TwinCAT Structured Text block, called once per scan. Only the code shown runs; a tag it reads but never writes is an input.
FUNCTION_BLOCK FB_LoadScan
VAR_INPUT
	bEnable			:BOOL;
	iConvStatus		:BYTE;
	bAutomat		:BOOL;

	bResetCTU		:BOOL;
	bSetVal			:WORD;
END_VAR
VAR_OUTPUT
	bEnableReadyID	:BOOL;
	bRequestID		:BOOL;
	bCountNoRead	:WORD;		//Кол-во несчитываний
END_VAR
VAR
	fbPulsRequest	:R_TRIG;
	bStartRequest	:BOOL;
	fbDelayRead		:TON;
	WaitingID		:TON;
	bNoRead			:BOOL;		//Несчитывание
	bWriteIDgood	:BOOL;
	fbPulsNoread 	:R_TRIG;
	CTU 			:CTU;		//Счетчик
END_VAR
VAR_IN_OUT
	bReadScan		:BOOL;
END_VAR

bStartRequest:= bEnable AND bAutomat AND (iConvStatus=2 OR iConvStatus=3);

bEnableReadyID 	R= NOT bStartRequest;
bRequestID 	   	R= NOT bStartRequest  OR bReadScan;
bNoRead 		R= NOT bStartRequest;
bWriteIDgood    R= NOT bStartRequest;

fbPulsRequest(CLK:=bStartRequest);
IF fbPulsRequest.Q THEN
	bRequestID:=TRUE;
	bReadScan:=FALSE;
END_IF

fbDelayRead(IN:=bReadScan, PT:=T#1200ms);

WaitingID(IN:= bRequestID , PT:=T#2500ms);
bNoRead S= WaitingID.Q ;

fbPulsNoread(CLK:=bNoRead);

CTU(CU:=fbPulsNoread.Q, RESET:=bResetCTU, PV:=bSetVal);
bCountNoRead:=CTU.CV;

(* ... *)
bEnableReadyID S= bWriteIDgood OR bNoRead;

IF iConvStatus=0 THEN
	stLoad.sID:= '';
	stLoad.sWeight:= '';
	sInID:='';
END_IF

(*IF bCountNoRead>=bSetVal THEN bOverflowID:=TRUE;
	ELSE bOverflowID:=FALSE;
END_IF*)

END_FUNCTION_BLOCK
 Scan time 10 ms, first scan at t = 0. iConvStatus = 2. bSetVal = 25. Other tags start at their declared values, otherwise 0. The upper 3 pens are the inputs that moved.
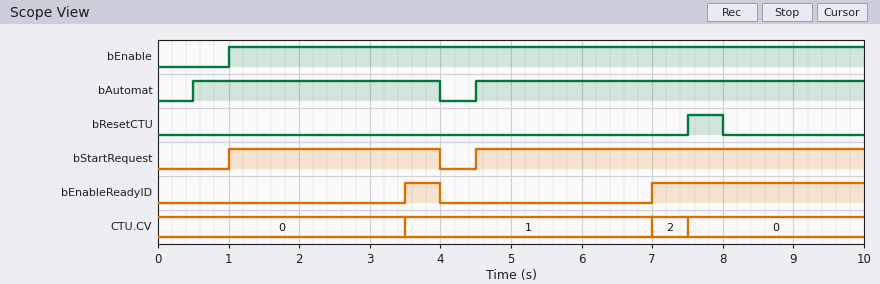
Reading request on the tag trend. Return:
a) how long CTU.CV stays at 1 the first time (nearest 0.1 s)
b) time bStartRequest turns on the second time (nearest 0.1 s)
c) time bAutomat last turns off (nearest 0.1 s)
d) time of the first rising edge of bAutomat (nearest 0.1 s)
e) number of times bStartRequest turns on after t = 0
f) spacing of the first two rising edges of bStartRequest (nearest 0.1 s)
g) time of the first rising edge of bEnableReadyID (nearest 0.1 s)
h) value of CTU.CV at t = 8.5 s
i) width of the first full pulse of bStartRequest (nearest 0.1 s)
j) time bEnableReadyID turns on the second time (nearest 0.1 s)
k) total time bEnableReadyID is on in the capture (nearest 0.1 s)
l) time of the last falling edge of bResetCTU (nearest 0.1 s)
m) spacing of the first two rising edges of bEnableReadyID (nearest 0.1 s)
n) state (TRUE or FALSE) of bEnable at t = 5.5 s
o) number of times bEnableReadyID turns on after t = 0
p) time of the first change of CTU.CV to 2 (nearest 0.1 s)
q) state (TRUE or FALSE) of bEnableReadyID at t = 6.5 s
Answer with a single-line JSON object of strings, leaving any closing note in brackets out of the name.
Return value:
{"how long CTU.CV stays at 1 the first time": "3.5 s", "time bStartRequest turns on the second time": "4.5 s", "time bAutomat last turns off": "4.0 s", "time of the first rising edge of bAutomat": "0.5 s", "number of times bStartRequest turns on after t = 0": "2", "spacing of the first two rising edges of bStartRequest": "3.5 s", "time of the first rising edge of bEnableReadyID": "3.5 s", "value of CTU.CV at t = 8.5 s": "0", "width of the first full pulse of bStartRequest": "3.0 s", "time bEnableReadyID turns on the second time": "7.0 s", "total time bEnableReadyID is on in the capture": "3.5 s", "time of the last falling edge of bResetCTU": "8.0 s", "spacing of the first two rising edges of bEnableReadyID": "3.5 s", "state (TRUE or FALSE) of bEnable at t = 5.5 s": "TRUE", "number of times bEnableReadyID turns on after t = 0": "2", "time of the first change of CTU.CV to 2": "7.0 s", "state (TRUE or FALSE) of bEnableReadyID at t = 6.5 s": "FALSE"}
